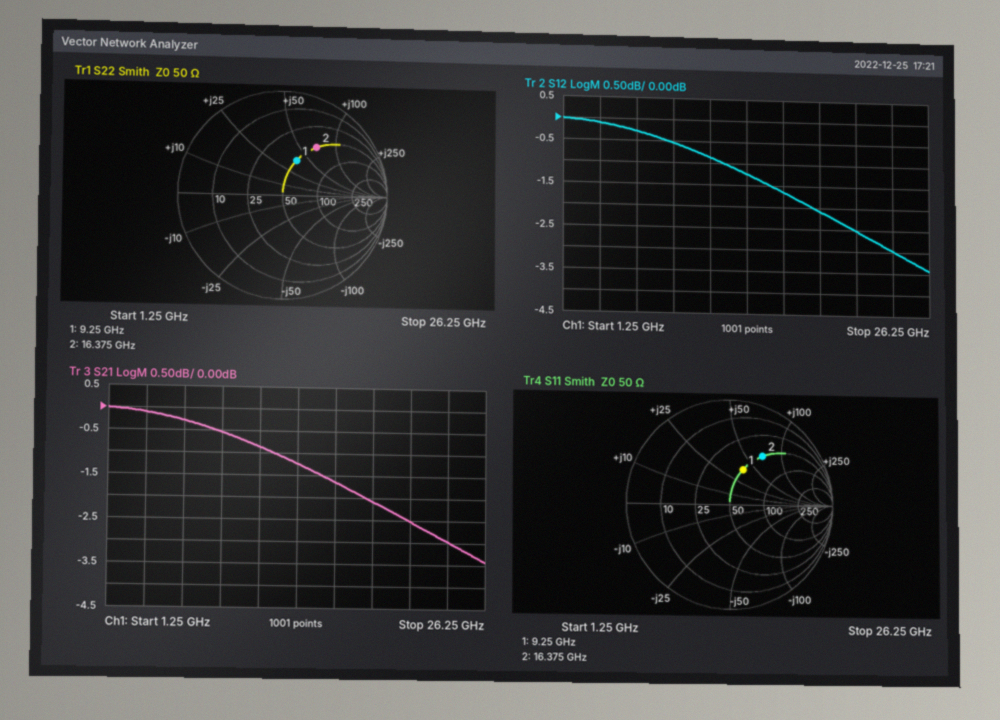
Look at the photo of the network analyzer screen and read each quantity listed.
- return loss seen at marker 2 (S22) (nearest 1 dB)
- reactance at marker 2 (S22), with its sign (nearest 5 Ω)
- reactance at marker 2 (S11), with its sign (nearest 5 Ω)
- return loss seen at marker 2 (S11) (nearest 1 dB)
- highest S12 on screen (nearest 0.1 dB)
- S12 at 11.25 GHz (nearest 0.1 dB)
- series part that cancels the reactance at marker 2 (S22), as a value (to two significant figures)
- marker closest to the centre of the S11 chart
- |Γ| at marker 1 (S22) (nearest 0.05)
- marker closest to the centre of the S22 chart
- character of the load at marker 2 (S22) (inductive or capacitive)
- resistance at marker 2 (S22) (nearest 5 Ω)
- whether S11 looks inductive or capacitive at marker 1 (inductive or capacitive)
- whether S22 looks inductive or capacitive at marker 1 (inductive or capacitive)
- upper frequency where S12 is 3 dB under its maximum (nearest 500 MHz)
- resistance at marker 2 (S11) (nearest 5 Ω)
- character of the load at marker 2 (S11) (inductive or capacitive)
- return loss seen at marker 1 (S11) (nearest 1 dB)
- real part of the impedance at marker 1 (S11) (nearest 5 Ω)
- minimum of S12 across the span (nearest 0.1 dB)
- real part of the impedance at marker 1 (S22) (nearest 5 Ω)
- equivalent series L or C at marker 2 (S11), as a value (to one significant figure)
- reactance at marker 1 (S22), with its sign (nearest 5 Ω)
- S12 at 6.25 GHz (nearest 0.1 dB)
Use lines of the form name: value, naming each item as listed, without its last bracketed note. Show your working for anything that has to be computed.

return loss seen at marker 2 (S22): 5 dB
reactance at marker 2 (S22), with its sign: +70 Ω
reactance at marker 2 (S11), with its sign: +70 Ω
return loss seen at marker 2 (S11): 5 dB
highest S12 on screen: 0.0 dB
S12 at 11.25 GHz: -0.9 dB
series part that cancels the reactance at marker 2 (S22), as a value: C = 1/(2π × 16.375 GHz × 70 Ω) ≈ 139 fF, so 140 fF to two significant figures
marker closest to the centre of the S11 chart: marker 1
|Γ| at marker 1 (S22): 0.35
marker closest to the centre of the S22 chart: marker 1
character of the load at marker 2 (S22): inductive
resistance at marker 2 (S22): 50 Ω
whether S11 looks inductive or capacitive at marker 1: inductive
whether S22 looks inductive or capacitive at marker 1: inductive
upper frequency where S12 is 3 dB under its maximum: 24.0 GHz
resistance at marker 2 (S11): 50 Ω
character of the load at marker 2 (S11): inductive
return loss seen at marker 1 (S11): 9 dB
real part of the impedance at marker 1 (S11): 50 Ω
minimum of S12 across the span: -3.4 dB
real part of the impedance at marker 1 (S22): 50 Ω
equivalent series L or C at marker 2 (S11), as a value: L = 70 Ω/(2π × 16.375 GHz) ≈ 680 pH, so 700 pH to one significant figure
reactance at marker 1 (S22), with its sign: +40 Ω
S12 at 6.25 GHz: -0.3 dB
